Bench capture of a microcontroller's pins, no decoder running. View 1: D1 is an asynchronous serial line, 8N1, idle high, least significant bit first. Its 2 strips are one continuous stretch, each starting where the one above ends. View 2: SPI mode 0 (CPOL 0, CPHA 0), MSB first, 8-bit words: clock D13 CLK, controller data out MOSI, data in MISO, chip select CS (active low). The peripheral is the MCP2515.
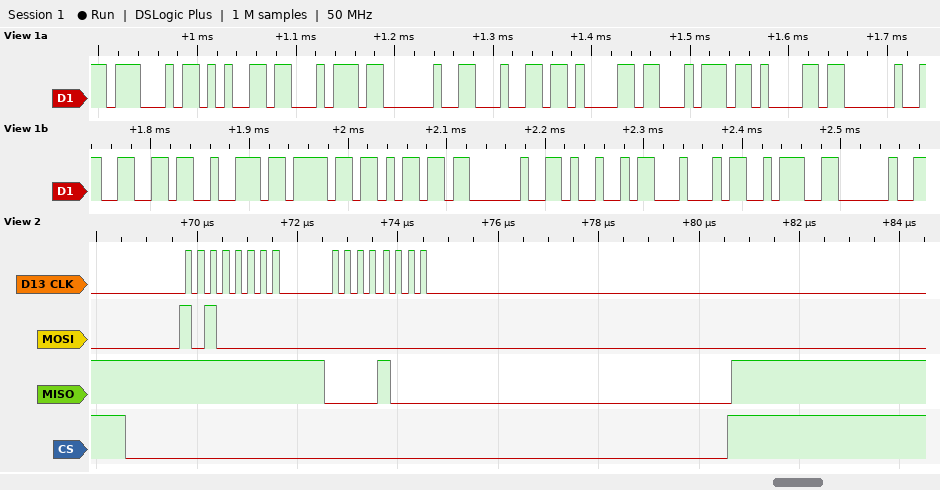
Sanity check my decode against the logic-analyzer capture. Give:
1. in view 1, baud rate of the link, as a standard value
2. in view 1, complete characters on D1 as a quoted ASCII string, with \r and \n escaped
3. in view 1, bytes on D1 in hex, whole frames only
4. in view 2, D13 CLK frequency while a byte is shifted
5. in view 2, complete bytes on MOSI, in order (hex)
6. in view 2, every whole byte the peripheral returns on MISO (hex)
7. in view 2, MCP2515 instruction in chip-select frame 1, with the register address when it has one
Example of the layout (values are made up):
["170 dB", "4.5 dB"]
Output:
["115200 baud", "\"Get data from ID: \"", "0x47 0x65 0x74 0x20 0x64 0x61 0x74 0x61 0x20 0x66 0x72 0x6F 0x6D 0x20 0x49 0x44 0x3A 0x20", "4 MHz", "A0 00", "FF 08", "READ STATUS"]
